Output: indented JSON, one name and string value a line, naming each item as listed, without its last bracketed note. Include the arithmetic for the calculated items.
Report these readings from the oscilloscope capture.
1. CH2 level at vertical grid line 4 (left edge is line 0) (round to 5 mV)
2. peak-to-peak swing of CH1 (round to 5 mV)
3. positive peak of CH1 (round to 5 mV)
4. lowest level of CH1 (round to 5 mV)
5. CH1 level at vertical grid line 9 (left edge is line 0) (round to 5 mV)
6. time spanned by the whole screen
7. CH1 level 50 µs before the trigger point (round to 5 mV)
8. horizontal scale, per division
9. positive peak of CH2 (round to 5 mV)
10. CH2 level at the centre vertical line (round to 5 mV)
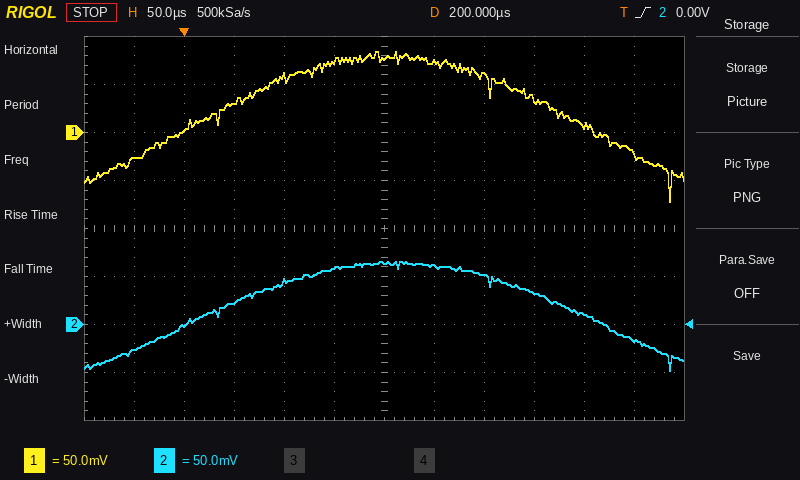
{
  "CH2 level at vertical grid line 4 (left edge is line 0)": "45 mV",
  "peak-to-peak swing of CH1": "85 mV − (-70 mV) = 155 mV",
  "positive peak of CH1": "85 mV",
  "lowest level of CH1": "-70 mV",
  "CH1 level at vertical grid line 9 (left edge is line 0)": "35 mV",
  "time spanned by the whole screen": "600 µs",
  "CH1 level 50 µs before the trigger point": "-25 mV",
  "horizontal scale, per division": "50 µs",
  "positive peak of CH2": "65 mV",
  "CH2 level at the centre vertical line": "65 mV"
}
